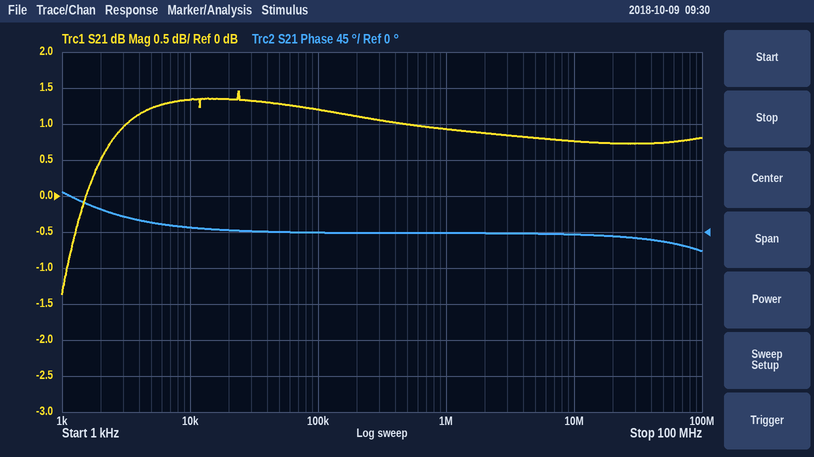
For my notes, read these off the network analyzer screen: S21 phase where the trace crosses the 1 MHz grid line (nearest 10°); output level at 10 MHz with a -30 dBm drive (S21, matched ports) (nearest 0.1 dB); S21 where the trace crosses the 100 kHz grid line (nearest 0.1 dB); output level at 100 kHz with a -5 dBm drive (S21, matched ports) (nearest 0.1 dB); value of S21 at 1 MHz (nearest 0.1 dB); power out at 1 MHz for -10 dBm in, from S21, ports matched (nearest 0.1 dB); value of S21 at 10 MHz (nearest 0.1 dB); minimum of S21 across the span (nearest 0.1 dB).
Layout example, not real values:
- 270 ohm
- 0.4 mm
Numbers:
- 0°
- -29.2 dBm
- 1.2 dB
- -3.8 dBm
- 0.9 dB
- -9.1 dBm
- 0.8 dB
- -1.4 dB
